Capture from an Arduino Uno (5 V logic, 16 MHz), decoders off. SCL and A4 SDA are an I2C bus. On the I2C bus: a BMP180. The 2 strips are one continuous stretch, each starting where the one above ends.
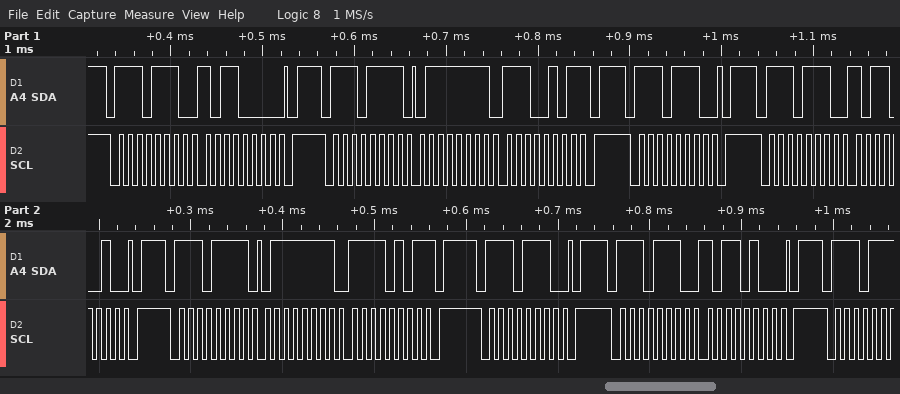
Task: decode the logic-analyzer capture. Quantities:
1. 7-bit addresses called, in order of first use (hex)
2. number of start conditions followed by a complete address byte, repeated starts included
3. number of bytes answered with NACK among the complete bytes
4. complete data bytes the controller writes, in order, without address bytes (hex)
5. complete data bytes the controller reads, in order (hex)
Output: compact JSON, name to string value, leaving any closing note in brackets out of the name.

{"7-bit addresses called, in order of first use": "0x77", "number of start conditions followed by a complete address byte, repeated starts included": "7", "number of bytes answered with NACK among the complete bytes": "2", "complete data bytes the controller writes, in order, without address bytes": "B0 B2 B4", "complete data bytes the controller reads, in order": "7F E5 7F F5"}
